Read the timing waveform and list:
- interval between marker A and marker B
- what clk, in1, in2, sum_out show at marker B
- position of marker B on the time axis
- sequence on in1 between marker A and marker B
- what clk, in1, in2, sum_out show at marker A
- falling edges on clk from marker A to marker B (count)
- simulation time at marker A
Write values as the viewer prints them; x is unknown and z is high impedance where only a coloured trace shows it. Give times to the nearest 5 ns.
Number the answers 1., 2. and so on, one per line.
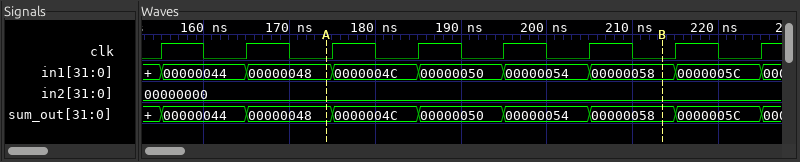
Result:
1. 40 ns
2. clk=0, in1=00000058, in2=00000000, sum_out=00000058
3. 215 ns
4. 00000048, 0000004C, 00000050, 00000054, 00000058
5. clk=0, in1=00000048, in2=00000000, sum_out=00000048
6. 4
7. 175 ns
